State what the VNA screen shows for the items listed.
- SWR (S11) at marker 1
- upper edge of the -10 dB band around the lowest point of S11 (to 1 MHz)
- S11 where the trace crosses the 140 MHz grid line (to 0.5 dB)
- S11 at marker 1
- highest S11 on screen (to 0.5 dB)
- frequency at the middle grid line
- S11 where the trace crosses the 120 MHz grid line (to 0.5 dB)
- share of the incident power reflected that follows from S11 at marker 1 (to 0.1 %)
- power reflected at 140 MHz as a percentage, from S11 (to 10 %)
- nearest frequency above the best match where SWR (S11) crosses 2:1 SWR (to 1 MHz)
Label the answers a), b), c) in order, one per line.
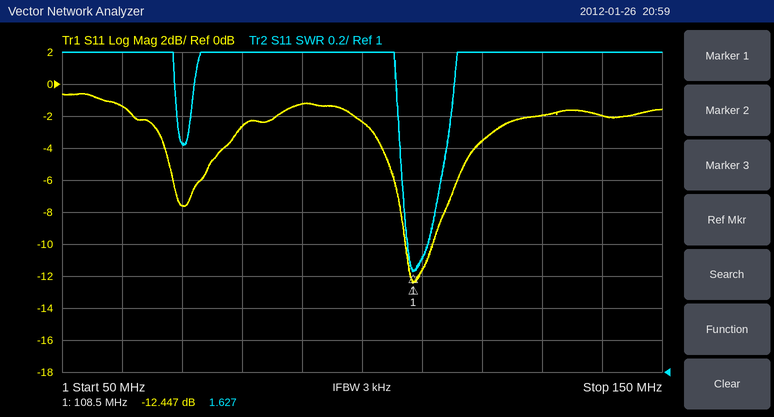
a) 1.627
b) 112 MHz
c) -2.0 dB
d) -12.447 dB
e) -0.5 dB
f) 100 MHz
g) -3.5 dB
h) 5.7 %
i) 60 %
j) 112 MHz
